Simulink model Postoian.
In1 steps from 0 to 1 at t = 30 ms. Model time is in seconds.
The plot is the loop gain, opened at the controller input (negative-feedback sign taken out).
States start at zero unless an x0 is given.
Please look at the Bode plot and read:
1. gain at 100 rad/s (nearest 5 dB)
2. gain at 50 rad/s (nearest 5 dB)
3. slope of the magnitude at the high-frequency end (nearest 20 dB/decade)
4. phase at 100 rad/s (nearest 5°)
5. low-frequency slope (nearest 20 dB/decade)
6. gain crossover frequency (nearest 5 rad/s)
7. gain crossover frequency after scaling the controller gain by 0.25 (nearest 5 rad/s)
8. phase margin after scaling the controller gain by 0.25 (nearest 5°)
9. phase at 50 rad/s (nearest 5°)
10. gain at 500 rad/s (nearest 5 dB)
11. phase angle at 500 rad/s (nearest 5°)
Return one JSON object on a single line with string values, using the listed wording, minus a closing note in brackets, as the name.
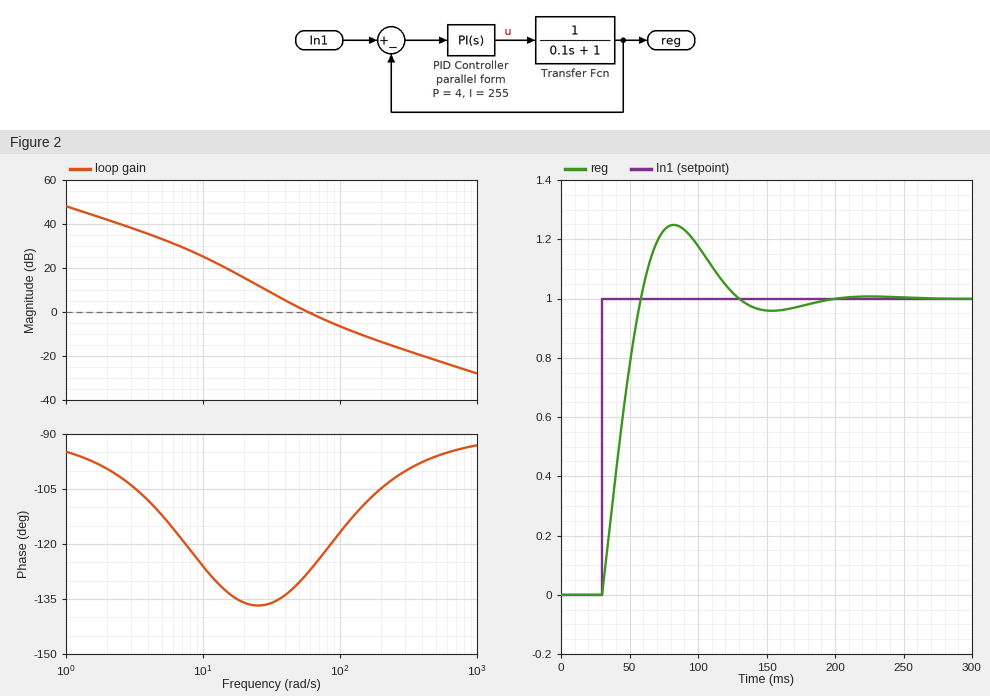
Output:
{"gain at 100 rad/s": "-5 dB", "gain at 50 rad/s": "0 dB", "slope of the magnitude at the high-frequency end": "-20 dB/decade", "phase at 100 rad/s": "-115°", "low-frequency slope": "-20 dB/decade", "gain crossover frequency": "60 rad/s", "gain crossover frequency after scaling the controller gain by 0.25": "25 rad/s", "phase margin after scaling the controller gain by 0.25": "45°", "phase at 50 rad/s": "-130°", "gain at 500 rad/s": "-20 dB", "phase angle at 500 rad/s": "-95°"}
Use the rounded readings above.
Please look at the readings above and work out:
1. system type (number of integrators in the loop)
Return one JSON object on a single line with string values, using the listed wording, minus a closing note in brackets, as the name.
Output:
{"system type": "1"}
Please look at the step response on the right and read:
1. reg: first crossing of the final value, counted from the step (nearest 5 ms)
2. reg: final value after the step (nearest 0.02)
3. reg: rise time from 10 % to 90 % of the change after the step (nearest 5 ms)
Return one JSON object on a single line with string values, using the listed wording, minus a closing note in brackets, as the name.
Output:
{"reg: first crossing of the final value, counted from the step": "30 ms", "reg: final value after the step": "1.00", "reg: rise time from 10 % to 90 % of the change after the step": "20 ms"}
